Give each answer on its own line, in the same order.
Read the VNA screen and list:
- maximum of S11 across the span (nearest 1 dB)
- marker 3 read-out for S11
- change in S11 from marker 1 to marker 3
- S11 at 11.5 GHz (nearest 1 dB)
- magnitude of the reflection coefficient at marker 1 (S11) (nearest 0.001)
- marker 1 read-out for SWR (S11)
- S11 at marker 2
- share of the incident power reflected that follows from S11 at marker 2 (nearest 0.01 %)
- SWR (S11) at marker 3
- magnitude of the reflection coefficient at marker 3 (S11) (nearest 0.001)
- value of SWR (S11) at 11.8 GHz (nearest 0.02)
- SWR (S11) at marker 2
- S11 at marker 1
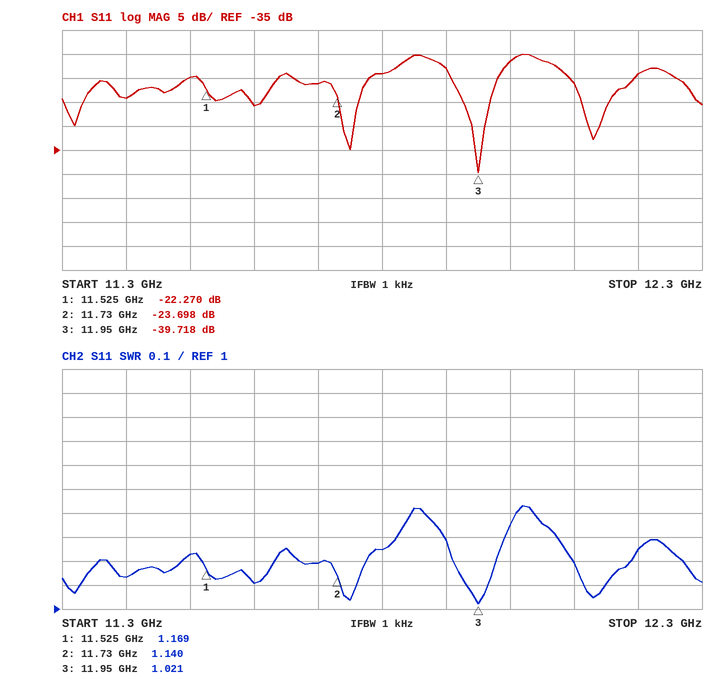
-15 dB
-39.718 dB
-17.448 dB
-20 dB
0.077
1.169
-23.698 dB
0.43 %
1.021
0.010
1.24
1.140
-22.270 dB
